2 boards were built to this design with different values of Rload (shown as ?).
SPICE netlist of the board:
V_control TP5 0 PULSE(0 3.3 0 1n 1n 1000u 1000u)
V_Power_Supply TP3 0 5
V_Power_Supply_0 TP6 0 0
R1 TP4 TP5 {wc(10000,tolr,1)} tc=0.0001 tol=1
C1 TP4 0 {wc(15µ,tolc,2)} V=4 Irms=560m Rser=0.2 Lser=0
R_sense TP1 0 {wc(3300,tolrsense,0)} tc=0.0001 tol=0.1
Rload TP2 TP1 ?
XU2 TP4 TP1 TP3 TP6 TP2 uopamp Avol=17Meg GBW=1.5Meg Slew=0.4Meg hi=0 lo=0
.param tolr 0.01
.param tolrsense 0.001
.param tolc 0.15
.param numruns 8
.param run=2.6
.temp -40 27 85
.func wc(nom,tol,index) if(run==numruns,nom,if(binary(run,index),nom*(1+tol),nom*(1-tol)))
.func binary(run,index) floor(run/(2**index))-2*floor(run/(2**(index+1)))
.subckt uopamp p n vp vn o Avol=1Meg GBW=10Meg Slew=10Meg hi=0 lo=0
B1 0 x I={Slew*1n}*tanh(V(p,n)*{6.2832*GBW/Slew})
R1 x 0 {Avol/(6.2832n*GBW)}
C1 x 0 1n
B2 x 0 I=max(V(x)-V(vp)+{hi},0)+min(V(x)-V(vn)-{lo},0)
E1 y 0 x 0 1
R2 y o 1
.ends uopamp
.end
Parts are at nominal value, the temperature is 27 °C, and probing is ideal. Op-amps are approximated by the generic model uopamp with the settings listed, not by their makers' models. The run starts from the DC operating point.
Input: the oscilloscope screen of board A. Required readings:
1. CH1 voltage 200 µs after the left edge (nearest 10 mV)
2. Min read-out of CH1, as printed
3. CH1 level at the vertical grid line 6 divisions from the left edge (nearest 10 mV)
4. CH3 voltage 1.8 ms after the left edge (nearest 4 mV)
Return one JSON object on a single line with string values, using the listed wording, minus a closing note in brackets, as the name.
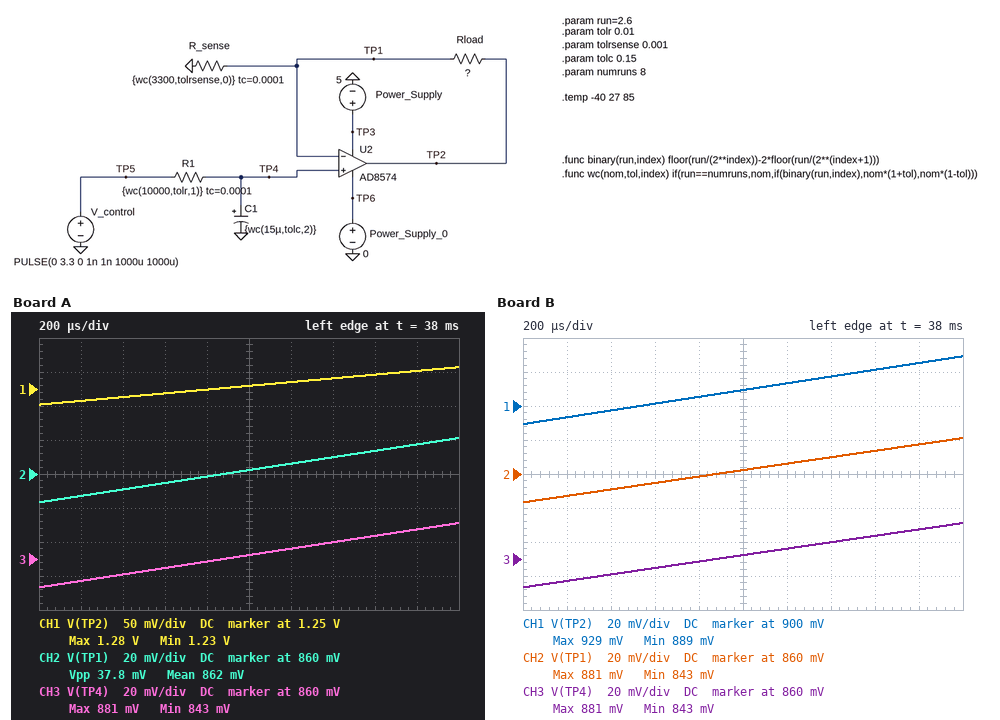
{"CH1 voltage 200 µs after the left edge": "1.23 V", "Min read-out of CH1, as printed": "1.23 V", "CH1 level at the vertical grid line 6 divisions from the left edge": "1.26 V", "CH3 voltage 1.8 ms after the left edge": "876 mV"}
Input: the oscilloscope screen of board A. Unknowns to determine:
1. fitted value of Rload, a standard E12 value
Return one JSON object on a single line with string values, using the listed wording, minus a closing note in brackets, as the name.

{"fitted value of Rload, a standard E12 value": "1.5 kΩ"}
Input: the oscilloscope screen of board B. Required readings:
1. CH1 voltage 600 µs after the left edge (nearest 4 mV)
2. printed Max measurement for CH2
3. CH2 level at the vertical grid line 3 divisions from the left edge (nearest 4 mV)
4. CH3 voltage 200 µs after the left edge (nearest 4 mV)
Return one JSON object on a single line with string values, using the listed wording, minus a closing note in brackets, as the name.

{"CH1 voltage 600 µs after the left edge": "900 mV", "printed Max measurement for CH2": "881 mV", "CH2 level at the vertical grid line 3 divisions from the left edge": "856 mV", "CH3 voltage 200 µs after the left edge": "848 mV"}
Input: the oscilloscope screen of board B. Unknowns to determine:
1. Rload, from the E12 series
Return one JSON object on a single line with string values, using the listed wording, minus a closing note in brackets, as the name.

{"Rload, from the E12 series": "180 Ω"}
